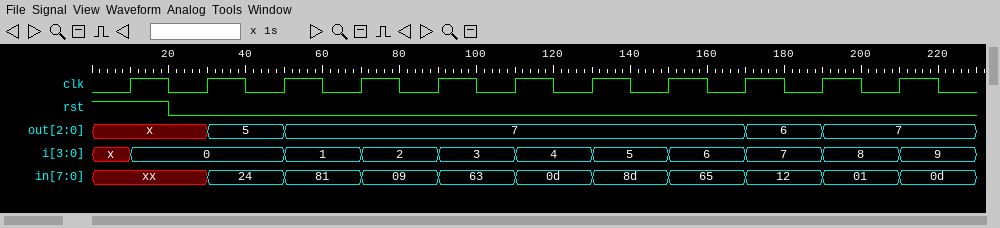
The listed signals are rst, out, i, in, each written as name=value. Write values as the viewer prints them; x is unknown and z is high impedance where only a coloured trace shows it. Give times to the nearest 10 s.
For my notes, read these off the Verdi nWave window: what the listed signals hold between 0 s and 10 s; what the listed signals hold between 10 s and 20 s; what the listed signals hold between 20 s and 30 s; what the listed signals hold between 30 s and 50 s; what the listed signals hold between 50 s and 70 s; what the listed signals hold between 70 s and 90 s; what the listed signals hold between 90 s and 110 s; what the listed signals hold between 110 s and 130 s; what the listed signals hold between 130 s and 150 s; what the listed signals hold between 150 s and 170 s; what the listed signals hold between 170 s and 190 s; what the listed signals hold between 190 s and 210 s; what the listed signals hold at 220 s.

rst=1, out=x, i=x, in=xx
rst=1, out=x, i=0, in=xx
rst=0, out=x, i=0, in=xx
rst=0, out=5, i=0, in=24
rst=0, out=7, i=1, in=81
rst=0, out=7, i=2, in=09
rst=0, out=7, i=3, in=63
rst=0, out=7, i=4, in=0d
rst=0, out=7, i=5, in=8d
rst=0, out=7, i=6, in=65
rst=0, out=6, i=7, in=12
rst=0, out=7, i=8, in=01
rst=0, out=7, i=9, in=0d
